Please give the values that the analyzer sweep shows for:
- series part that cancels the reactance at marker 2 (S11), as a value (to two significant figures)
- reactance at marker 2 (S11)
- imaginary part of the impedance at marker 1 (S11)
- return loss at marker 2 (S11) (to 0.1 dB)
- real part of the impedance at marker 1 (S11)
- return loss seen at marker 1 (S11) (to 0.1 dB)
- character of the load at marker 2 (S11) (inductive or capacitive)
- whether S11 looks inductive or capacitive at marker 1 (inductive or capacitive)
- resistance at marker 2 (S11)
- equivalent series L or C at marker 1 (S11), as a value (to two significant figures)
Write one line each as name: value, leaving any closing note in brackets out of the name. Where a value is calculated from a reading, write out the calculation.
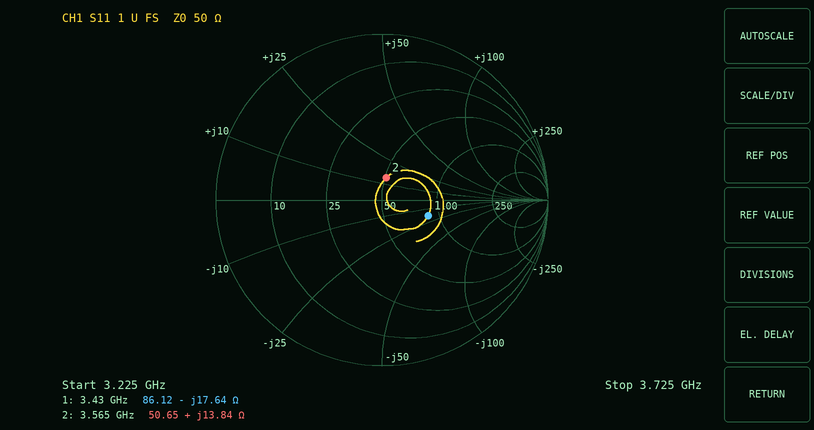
series part that cancels the reactance at marker 2 (S11), as a value: C = 1/(2π × 3.565 GHz × 13.84 Ω) ≈ 3.2 pF
reactance at marker 2: +13.84 Ω
imaginary part of the impedance at marker 1: -17.64 Ω
return loss at marker 2 (S11): 17.3 dB
real part of the impedance at marker 1: 86.12 Ω
return loss seen at marker 1 (S11): 10.7 dB
character of the load at marker 2 (S11): inductive
whether S11 looks inductive or capacitive at marker 1: capacitive
resistance at marker 2: 50.65 Ω
equivalent series L or C at marker 1 (S11), as a value: C = 1/(2π × 3.43 GHz × 17.64 Ω) ≈ 2.6 pF
